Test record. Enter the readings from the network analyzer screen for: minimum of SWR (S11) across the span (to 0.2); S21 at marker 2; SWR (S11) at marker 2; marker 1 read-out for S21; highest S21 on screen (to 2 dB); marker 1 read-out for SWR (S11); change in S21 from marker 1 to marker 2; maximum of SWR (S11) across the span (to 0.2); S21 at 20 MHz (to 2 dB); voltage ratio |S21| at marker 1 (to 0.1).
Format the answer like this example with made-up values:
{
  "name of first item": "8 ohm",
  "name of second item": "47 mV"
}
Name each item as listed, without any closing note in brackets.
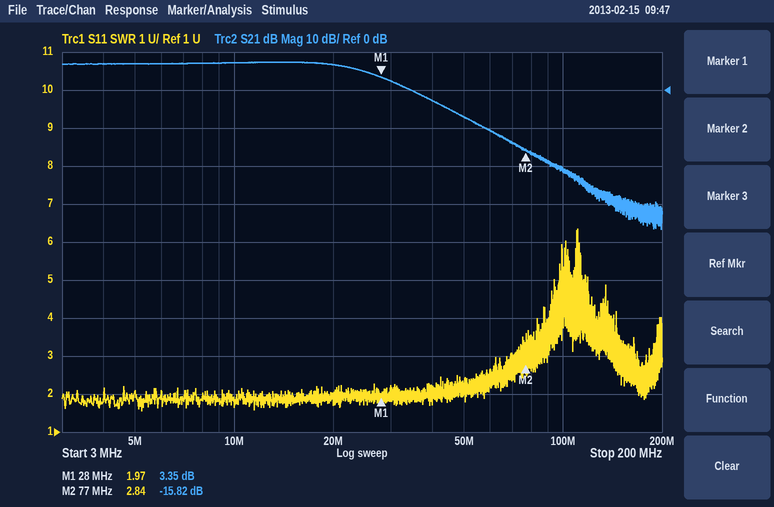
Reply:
{
  "minimum of SWR (S11) across the span": "1.6",
  "S21 at marker 2": "-15.82 dB",
  "SWR (S11) at marker 2": "2.84",
  "marker 1 read-out for S21": "3.35 dB",
  "highest S21 on screen": "8 dB",
  "marker 1 read-out for SWR": "1.97",
  "change in S21 from marker 1 to marker 2": "-19.17 dB",
  "maximum of SWR (S11) across the span": "6.4",
  "S21 at 20 MHz": "6 dB",
  "voltage ratio |S21| at marker 1": "1.5"
}
